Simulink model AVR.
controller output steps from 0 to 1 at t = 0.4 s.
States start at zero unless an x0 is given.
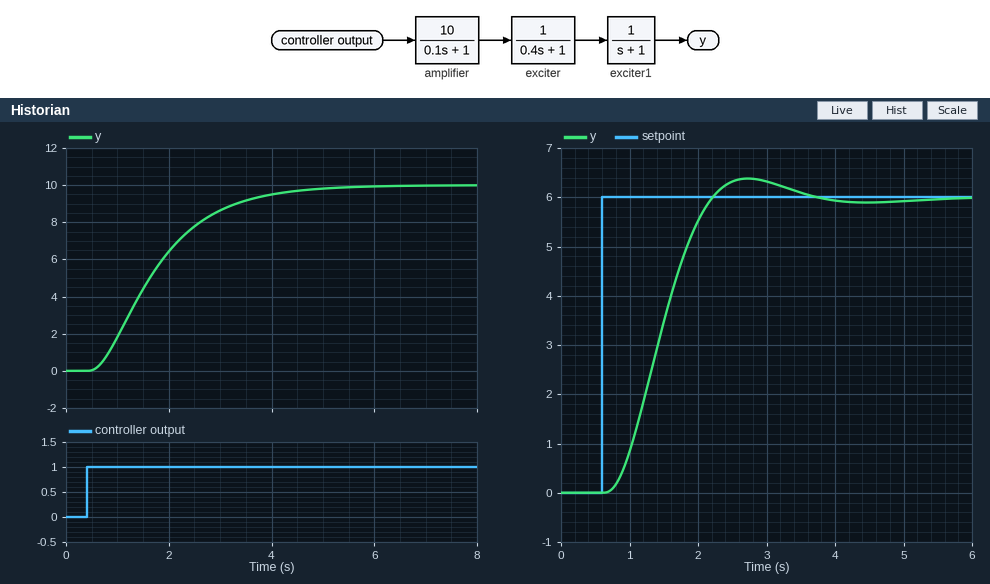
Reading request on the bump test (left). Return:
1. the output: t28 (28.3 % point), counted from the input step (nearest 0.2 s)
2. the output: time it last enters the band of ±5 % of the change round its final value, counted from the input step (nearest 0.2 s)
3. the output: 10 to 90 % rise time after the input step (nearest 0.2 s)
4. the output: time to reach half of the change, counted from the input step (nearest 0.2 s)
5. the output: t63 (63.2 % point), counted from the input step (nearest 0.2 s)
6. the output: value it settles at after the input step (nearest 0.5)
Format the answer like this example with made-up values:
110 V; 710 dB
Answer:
0.8 s; 3.6 s; 2.4 s; 1.2 s; 1.6 s; 10.0
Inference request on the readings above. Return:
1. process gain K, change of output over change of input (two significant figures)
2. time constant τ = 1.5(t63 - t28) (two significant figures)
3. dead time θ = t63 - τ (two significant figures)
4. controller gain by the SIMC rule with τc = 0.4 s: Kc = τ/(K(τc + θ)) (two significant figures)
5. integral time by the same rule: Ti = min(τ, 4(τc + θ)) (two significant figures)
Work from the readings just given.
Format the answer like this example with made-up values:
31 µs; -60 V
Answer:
10; 1.2 s; 0.40 s; 0.15; 1.2 s
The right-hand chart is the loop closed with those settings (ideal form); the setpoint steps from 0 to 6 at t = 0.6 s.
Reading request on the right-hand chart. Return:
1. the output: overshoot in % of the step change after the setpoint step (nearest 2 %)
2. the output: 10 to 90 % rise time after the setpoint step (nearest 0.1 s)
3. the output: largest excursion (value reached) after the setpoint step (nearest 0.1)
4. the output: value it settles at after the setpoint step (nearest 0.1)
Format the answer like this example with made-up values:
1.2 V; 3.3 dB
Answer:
6 %; 1.0 s; 6.4; 6.0
